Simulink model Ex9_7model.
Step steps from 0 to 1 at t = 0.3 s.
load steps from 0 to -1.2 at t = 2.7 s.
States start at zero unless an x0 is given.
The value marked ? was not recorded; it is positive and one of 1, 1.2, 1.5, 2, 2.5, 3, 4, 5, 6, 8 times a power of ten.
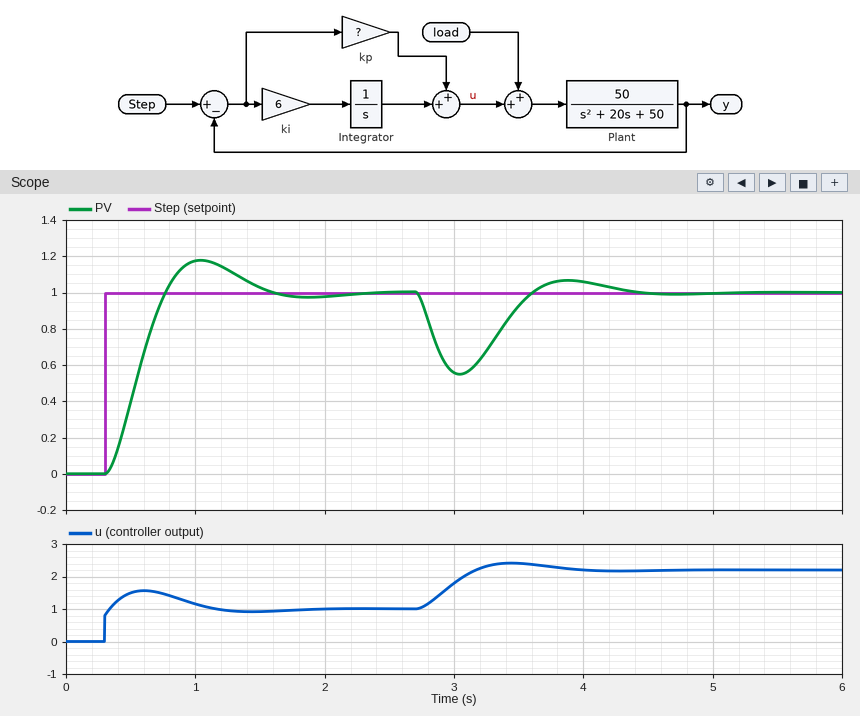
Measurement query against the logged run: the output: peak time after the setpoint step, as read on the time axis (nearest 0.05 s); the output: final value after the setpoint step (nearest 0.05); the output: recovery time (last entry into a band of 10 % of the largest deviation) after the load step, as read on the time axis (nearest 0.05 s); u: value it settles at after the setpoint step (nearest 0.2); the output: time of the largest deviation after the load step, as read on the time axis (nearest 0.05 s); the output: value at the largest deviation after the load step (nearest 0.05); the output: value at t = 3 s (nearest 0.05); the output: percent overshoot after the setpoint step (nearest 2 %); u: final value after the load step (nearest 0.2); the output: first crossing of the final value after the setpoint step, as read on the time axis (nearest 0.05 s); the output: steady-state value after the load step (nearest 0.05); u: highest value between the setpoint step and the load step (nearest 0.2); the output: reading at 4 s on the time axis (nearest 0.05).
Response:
1.05 s
1.00
4.10 s
1.0
3.05 s
0.55
0.55
18 %
2.2
0.75 s
1.00
1.6
1.05
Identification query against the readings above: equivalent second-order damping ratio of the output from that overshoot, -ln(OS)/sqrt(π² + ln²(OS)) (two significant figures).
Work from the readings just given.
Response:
0.48
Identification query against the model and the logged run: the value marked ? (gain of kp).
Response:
0.8
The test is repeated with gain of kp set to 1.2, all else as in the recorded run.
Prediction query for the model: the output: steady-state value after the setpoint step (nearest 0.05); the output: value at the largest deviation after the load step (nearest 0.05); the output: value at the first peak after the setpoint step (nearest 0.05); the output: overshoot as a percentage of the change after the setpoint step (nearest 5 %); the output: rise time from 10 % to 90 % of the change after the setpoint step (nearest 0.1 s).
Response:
1.00
0.60
1.10
10 %
0.3 s
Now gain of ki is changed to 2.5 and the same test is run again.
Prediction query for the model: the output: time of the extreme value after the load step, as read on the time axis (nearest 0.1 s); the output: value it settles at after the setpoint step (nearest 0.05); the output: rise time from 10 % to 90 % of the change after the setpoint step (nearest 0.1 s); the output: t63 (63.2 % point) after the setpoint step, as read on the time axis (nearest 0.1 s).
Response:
3.1 s
1.00
0.7 s
0.7 s
